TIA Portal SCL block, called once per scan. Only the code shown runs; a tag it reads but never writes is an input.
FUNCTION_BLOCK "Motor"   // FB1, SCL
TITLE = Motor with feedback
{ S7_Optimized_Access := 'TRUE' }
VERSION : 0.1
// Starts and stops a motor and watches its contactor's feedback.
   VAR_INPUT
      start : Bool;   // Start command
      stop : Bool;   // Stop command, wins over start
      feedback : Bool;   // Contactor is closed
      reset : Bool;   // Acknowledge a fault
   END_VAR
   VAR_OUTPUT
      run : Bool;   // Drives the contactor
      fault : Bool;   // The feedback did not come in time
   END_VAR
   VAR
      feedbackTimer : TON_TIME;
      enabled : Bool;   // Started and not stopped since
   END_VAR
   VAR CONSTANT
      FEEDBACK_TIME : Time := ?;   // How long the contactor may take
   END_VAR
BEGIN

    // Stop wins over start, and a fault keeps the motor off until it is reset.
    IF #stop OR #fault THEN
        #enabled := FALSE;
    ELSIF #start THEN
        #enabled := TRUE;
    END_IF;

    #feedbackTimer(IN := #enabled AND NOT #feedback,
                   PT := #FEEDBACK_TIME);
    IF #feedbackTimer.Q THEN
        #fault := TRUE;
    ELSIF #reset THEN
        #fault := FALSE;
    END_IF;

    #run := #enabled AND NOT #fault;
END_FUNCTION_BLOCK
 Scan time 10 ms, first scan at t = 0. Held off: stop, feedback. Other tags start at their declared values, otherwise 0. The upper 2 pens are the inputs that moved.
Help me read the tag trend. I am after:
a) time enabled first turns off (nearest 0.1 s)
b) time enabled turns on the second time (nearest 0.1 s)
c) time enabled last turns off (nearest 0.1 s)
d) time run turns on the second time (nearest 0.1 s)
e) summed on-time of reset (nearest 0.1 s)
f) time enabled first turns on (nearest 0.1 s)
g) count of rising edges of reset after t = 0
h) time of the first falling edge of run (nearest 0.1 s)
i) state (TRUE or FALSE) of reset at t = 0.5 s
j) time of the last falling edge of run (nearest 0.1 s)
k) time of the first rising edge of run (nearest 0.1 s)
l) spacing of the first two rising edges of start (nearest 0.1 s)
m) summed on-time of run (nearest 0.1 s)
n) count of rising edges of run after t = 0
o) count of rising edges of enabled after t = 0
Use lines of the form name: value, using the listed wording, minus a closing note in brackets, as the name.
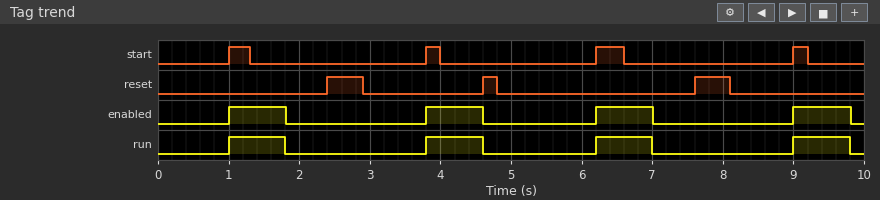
time enabled first turns off: 1.8 s
time enabled turns on the second time: 3.8 s
time enabled last turns off: 9.8 s
time run turns on the second time: 3.8 s
summed on-time of reset: 1.2 s
time enabled first turns on: 1.0 s
count of rising edges of reset after t = 0: 3
time of the first falling edge of run: 1.8 s
state (TRUE or FALSE) of reset at t = 0.5 s: FALSE
time of the last falling edge of run: 9.8 s
time of the first rising edge of run: 1.0 s
spacing of the first two rising edges of start: 2.8 s
summed on-time of run: 3.2 s
count of rising edges of run after t = 0: 4
count of rising edges of enabled after t = 0: 4
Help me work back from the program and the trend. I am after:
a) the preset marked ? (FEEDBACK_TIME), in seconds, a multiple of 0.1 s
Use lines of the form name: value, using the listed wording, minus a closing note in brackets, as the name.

the preset marked ? (FEEDBACK_TIME), in seconds, a multiple of 0.1 s: 0.8 s
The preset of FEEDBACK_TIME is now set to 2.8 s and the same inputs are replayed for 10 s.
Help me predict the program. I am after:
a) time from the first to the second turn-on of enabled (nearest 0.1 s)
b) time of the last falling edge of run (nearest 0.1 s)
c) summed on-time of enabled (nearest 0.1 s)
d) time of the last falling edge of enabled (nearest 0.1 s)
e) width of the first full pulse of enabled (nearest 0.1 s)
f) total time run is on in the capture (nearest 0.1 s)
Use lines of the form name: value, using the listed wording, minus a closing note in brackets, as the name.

time from the first to the second turn-on of enabled: 5.2 s
time of the last falling edge of run: 9.0 s
summed on-time of enabled: 5.6 s
time of the last falling edge of enabled: 9.0 s
width of the first full pulse of enabled: 2.8 s
total time run is on in the capture: 5.6 s
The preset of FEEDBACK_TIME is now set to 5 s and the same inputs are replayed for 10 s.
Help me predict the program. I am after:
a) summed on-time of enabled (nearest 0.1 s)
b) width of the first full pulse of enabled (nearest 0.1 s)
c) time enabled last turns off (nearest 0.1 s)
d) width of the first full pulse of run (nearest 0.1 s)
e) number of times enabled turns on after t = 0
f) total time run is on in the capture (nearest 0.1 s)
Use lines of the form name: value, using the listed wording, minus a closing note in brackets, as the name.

summed on-time of enabled: 6.0 s
width of the first full pulse of enabled: 5.0 s
time enabled last turns off: 6.0 s
width of the first full pulse of run: 5.0 s
number of times enabled turns on after t = 0: 2
total time run is on in the capture: 6.0 s
